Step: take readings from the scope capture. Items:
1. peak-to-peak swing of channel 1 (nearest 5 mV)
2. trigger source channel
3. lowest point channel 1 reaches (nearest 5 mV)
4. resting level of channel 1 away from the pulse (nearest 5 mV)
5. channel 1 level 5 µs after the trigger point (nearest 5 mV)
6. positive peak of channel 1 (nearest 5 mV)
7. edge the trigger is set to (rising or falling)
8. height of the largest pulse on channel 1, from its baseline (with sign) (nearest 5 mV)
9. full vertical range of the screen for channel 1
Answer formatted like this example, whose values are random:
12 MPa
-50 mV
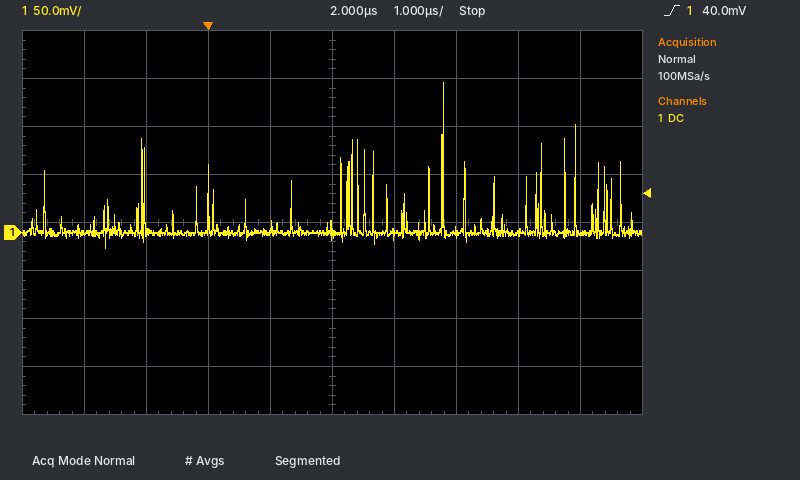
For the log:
170 mV
channel 1
-15 mV
0 mV
0 mV
155 mV
rising
+155 mV
400 mV
